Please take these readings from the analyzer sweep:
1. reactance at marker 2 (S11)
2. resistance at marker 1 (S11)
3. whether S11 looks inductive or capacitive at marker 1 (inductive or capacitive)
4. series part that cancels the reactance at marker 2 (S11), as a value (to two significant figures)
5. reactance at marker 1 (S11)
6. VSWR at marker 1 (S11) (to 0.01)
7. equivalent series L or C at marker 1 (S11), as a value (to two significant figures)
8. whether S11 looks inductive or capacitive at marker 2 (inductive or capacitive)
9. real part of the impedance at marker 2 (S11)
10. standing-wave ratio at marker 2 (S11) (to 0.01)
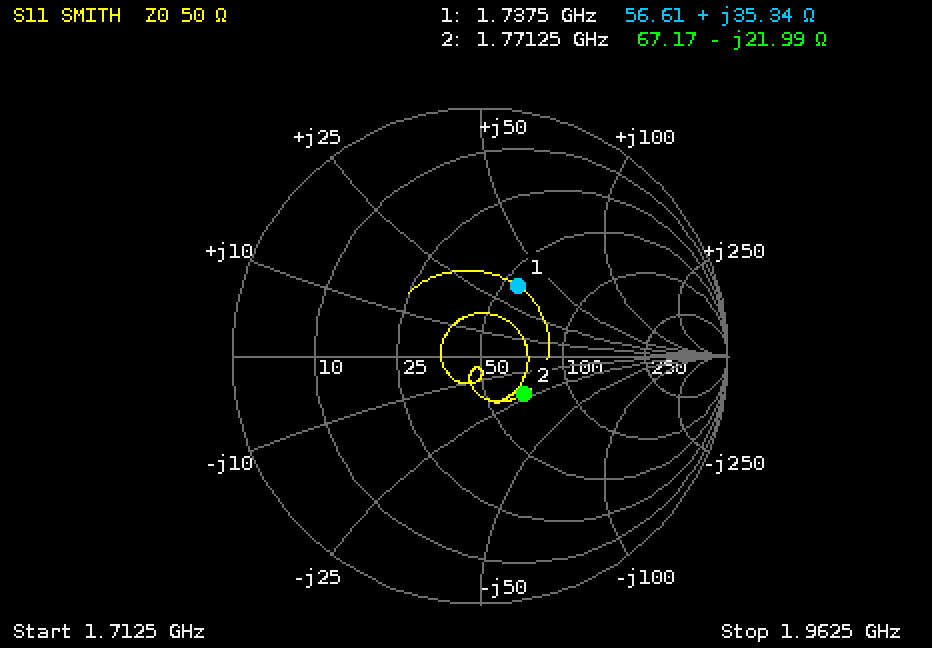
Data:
-21.99 Ω
56.61 Ω
inductive
2.0 nH
+35.34 Ω
1.94
3.2 nH
capacitive
67.17 Ω
1.61
